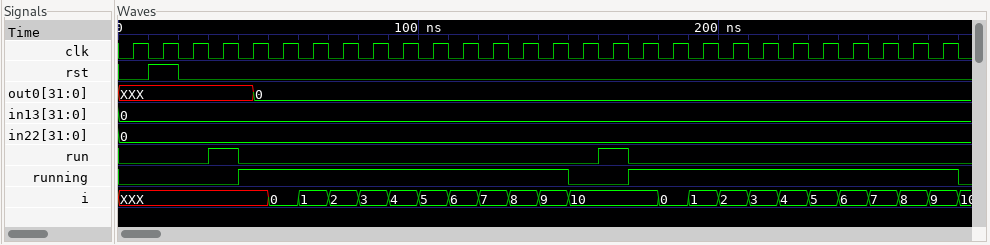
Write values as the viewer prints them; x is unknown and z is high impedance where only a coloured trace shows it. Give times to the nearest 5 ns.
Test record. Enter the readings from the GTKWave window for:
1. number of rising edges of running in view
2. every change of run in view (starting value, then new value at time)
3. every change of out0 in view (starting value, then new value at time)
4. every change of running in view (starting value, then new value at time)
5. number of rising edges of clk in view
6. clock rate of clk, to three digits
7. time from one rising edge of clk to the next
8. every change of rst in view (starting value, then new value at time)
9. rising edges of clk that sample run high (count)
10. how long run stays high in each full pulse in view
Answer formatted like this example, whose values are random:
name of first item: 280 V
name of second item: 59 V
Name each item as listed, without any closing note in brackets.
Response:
number of rising edges of running in view: 2
every change of run in view: 0, 1 at 30 ns, 0 at 40 ns, 1 at 160 ns, 0 at 170 ns
every change of out0 in view: XXX, 0 at 45 ns
every change of running in view: 0, 1 at 40 ns, 0 at 150 ns, 1 at 170 ns, 0 at 280 ns
number of rising edges of clk in view: 28
clock rate of clk, to three digits: 100 MHz
time from one rising edge of clk to the next: 10 ns
every change of rst in view: 0, 1 at 10 ns, 0 at 20 ns
rising edges of clk that sample run high: 2
how long run stays high in each full pulse in view: 10 ns, 10 ns
